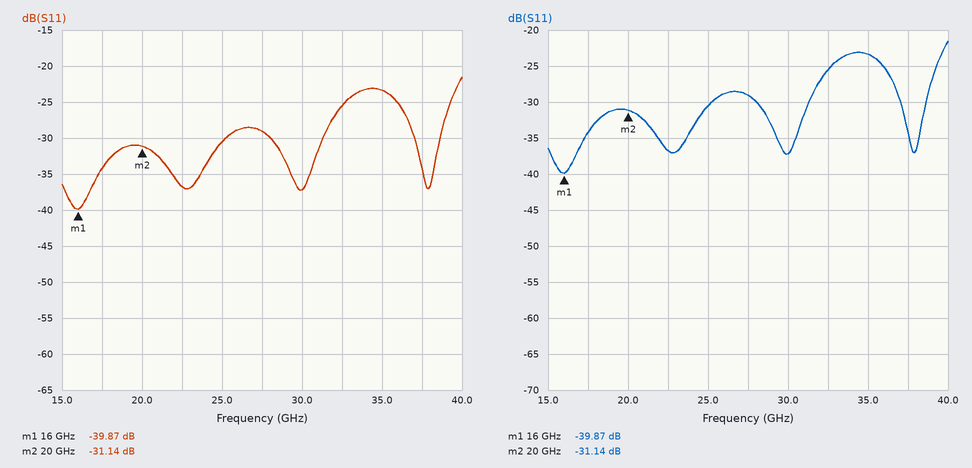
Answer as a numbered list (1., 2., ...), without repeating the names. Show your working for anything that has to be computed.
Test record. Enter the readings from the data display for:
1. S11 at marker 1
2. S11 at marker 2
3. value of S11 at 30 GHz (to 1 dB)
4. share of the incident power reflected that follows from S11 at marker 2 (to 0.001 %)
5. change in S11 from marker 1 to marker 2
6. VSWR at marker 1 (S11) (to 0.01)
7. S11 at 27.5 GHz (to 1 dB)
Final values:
1. -39.87 dB
2. -31.14 dB
3. -37 dB
4. 10^(-31.14/10) ≈ 0.077 %
5. -31.14 − (-39.87) = 8.73 dB
6. (1 + 0.0102)/(1 − 0.0102) ≈ 1.02
7. -29 dB
